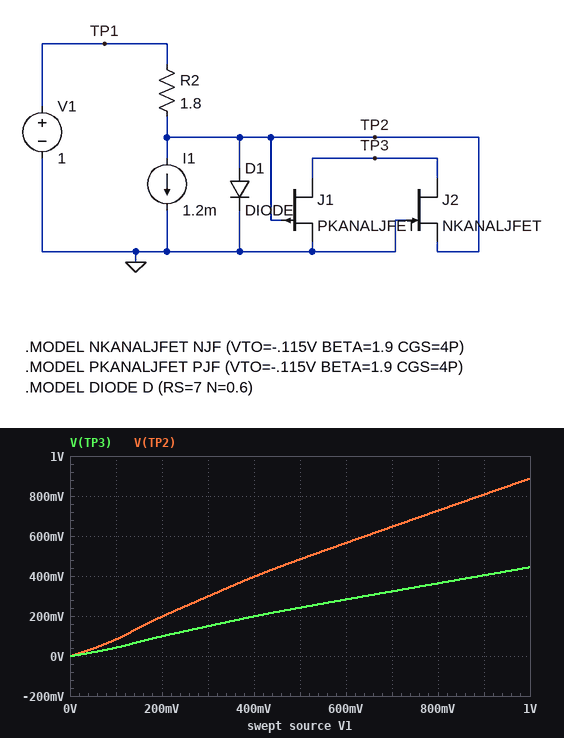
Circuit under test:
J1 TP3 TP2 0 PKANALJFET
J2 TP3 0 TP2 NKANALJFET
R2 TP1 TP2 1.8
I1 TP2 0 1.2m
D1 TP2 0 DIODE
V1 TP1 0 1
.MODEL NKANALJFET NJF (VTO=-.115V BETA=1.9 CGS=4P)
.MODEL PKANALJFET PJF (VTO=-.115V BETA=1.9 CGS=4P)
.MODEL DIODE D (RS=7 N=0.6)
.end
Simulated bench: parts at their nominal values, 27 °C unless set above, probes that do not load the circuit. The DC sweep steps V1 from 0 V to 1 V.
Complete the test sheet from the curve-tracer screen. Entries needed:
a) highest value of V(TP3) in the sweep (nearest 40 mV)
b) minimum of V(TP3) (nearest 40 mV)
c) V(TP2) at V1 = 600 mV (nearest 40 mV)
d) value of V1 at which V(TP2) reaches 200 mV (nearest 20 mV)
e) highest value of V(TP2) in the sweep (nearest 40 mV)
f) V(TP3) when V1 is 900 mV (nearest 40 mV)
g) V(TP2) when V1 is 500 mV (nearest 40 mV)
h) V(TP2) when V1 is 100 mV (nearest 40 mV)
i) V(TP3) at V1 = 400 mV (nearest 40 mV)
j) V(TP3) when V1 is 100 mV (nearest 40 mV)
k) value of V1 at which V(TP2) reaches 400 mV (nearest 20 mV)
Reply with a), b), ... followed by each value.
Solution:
a) 440 mV
b) 0 V
c) 560 mV
d) 200 mV
e) 880 mV
f) 400 mV
g) 480 mV
h) 80 mV
i) 200 mV
j) 40 mV
k) 400 mV
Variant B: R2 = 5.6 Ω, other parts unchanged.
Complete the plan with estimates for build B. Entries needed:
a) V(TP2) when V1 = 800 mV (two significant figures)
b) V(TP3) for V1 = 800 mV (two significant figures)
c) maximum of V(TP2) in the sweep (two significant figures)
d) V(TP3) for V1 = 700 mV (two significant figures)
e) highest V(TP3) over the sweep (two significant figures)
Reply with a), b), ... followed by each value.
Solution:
a) 640 mV
b) 320 mV
c) 750 mV
d) 290 mV
e) 380 mV
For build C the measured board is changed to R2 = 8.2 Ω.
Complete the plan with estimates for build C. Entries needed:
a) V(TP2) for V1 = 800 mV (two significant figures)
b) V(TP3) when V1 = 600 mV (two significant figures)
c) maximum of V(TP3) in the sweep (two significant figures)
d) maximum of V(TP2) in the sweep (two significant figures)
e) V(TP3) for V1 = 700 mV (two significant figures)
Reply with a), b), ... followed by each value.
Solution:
a) 600 mV
b) 250 mV
c) 350 mV
d) 700 mV
e) 280 mV
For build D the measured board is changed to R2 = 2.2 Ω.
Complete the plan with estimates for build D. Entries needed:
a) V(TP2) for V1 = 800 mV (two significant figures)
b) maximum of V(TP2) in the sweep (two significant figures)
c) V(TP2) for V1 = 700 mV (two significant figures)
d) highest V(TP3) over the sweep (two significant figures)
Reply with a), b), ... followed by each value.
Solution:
a) 710 mV
b) 870 mV
c) 640 mV
d) 430 mV
